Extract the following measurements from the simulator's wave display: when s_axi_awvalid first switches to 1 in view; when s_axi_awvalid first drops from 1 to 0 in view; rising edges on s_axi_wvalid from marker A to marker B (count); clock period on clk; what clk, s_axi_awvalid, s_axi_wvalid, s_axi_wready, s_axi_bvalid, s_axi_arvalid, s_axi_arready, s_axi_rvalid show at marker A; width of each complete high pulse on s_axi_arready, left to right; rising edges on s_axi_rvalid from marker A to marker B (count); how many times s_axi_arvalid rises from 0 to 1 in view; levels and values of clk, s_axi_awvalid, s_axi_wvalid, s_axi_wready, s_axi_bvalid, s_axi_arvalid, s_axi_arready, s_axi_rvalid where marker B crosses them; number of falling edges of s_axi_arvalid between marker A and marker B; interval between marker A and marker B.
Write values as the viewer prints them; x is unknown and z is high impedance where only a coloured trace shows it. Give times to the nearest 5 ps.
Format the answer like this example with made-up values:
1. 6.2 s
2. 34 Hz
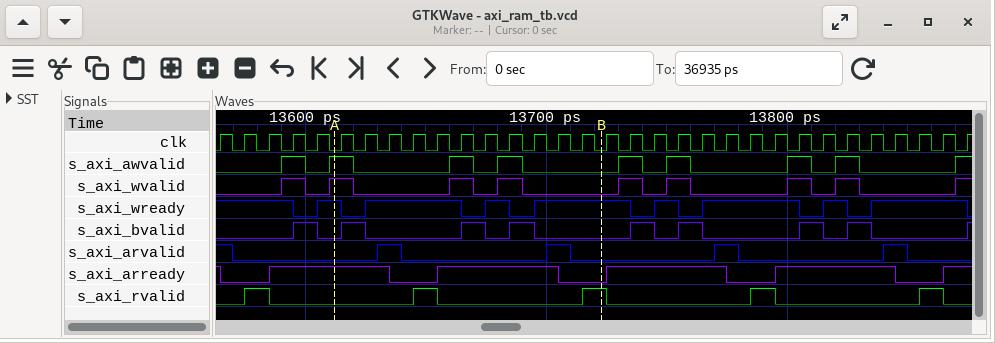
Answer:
1. 13590 ps
2. 13600 ps
3. 2
4. 10 ps
5. clk=0, s_axi_awvalid=1, s_axi_wvalid=1, s_axi_wready=1, s_axi_bvalid=0, s_axi_arvalid=0, s_axi_arready=1, s_axi_rvalid=0
6. 50 ps, 50 ps, 50 ps, 50 ps
7. 2
8. 4
9. clk=0, s_axi_awvalid=0, s_axi_wvalid=0, s_axi_wready=1, s_axi_bvalid=0, s_axi_arvalid=0, s_axi_arready=0, s_axi_rvalid=1
10. 2
11. 110 ps
